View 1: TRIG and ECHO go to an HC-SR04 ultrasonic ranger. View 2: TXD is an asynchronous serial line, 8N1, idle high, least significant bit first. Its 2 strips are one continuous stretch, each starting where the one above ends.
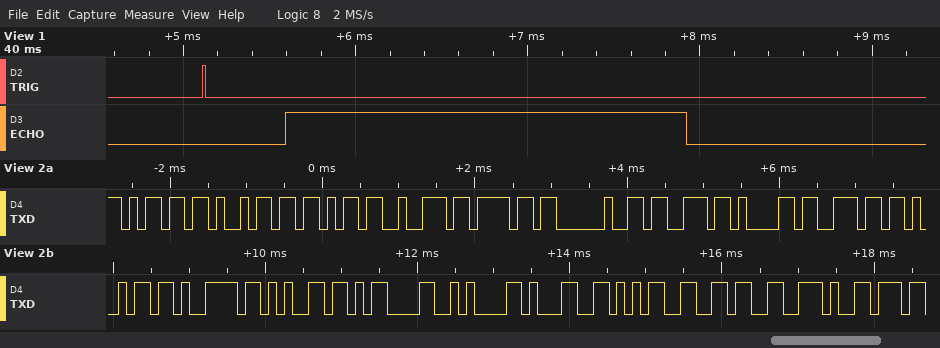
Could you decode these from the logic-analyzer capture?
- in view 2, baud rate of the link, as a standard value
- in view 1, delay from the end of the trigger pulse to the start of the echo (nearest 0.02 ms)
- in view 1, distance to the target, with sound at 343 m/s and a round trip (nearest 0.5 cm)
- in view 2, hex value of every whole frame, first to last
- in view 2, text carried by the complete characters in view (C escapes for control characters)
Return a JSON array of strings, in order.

["9600 baud", "0.46 ms", "40 cm", "6D 69 6B 72 6F 20 73 61 6E 69 79 65 0D 0A 31 35 36 2E", "\"mikro saniye\\r\\n156.\""]
